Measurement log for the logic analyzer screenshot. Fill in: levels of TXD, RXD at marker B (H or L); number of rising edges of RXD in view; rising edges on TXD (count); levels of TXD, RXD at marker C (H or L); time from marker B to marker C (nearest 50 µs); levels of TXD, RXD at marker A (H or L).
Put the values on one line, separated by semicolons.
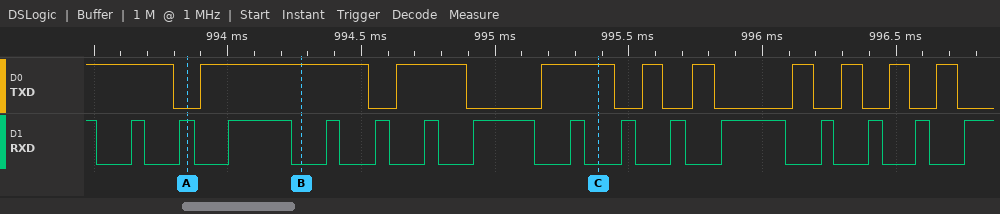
TXD=H, RXD=L; 15; 9; TXD=H, RXD=L; 1100 µs; TXD=L, RXD=H
